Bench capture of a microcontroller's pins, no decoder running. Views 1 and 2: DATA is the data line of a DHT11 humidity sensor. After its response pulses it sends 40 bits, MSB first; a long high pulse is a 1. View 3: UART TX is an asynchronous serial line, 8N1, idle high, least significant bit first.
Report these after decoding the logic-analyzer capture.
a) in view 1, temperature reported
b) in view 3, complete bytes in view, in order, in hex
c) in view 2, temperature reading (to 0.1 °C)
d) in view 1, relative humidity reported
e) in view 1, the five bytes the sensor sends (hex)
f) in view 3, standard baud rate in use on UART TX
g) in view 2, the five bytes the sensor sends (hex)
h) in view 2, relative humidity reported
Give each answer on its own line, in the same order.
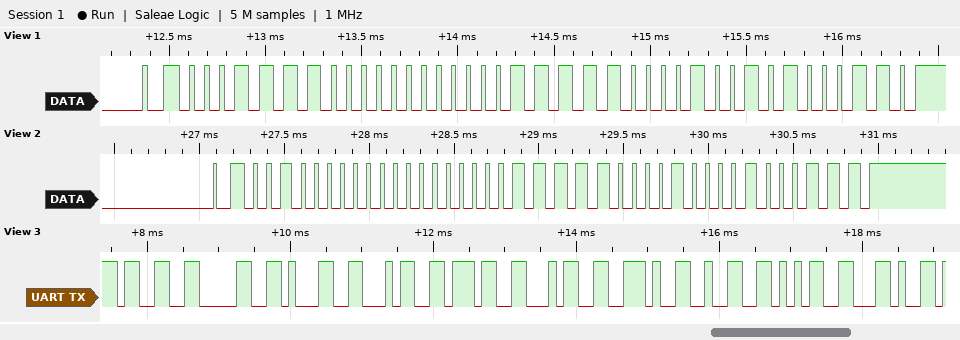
31.9 °C
33 30 31 34 37 34 2E 32 35 2C
31.8 °C
30 %
1E 00 1F 09 46
9600 baud
20 00 1F 08 47
32 %
